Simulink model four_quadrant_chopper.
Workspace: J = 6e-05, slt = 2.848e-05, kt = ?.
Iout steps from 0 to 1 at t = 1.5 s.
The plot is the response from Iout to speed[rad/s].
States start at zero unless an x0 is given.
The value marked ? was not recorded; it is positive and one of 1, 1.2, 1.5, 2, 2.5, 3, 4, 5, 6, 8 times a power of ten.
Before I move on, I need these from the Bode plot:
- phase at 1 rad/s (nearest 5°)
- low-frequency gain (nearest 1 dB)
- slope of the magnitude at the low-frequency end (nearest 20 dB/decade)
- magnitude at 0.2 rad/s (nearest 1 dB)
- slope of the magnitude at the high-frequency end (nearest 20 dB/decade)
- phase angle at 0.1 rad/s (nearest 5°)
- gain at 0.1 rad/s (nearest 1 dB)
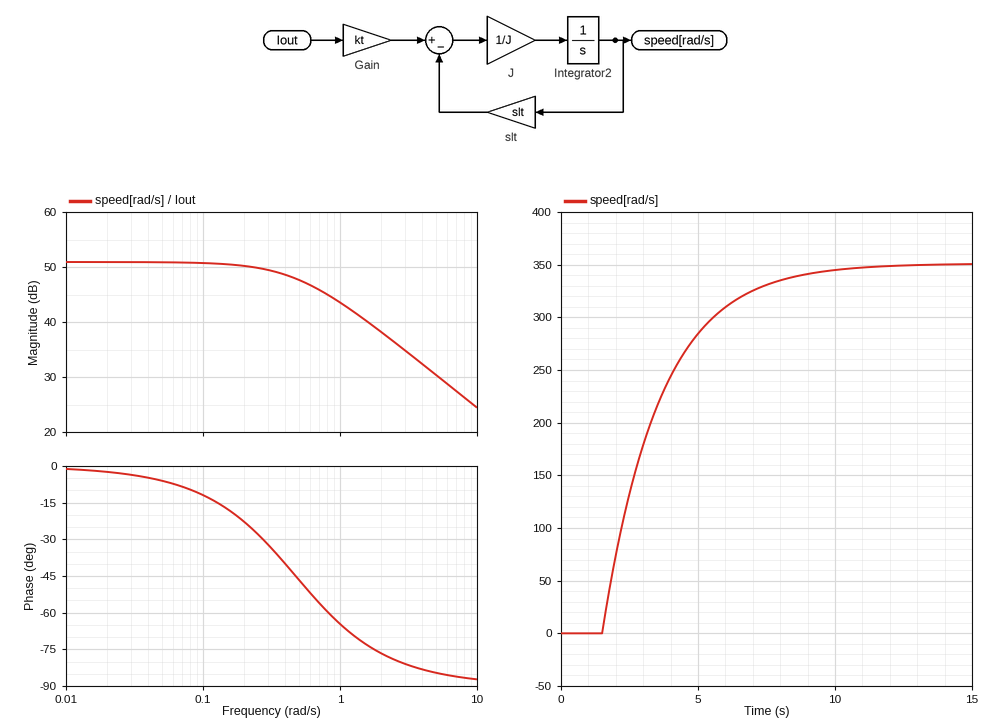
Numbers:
-65°
51 dB
0 dB/decade
50 dB
-20 dB/decade
-10°
51 dB
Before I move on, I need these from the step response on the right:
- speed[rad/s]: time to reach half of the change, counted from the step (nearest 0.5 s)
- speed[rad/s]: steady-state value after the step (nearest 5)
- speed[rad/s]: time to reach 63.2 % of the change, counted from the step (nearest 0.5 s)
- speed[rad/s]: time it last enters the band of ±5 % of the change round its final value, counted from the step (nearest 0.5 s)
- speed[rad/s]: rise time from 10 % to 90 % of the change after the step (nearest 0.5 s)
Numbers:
1.5 s
350
2.0 s
6.5 s
4.5 s
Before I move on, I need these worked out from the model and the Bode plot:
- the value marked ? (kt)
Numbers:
0.01
